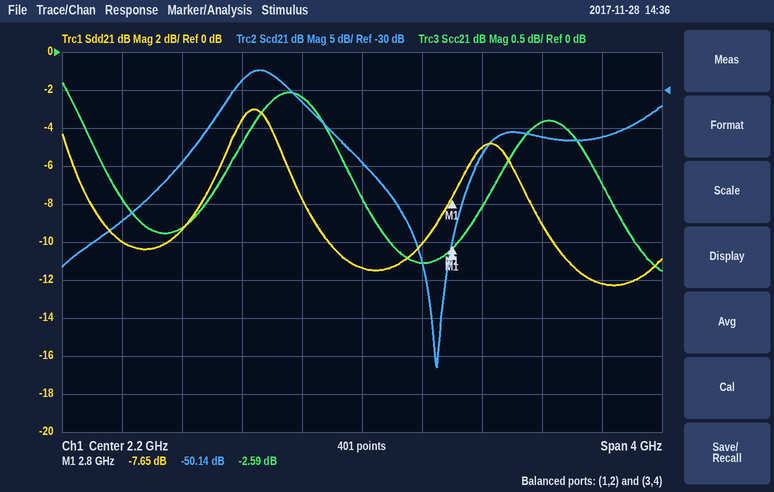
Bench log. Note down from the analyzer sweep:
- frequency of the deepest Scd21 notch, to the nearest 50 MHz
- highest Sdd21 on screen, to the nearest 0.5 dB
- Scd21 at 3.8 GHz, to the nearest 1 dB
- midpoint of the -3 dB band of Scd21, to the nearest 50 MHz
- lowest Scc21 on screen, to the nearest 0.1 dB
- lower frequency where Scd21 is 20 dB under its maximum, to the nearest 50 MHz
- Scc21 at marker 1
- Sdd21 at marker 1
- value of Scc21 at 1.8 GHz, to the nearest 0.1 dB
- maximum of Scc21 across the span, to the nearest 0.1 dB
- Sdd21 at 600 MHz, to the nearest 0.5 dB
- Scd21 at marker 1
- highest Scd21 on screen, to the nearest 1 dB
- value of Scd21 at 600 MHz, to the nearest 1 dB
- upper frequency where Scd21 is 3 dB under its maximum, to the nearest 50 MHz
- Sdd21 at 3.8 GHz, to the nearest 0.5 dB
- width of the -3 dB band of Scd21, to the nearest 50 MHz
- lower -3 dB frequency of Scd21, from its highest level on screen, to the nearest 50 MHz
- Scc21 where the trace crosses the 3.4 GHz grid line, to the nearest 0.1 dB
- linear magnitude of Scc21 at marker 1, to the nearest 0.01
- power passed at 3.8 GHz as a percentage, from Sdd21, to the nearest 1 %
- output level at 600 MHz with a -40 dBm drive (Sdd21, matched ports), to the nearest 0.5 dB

2.70 GHz
-3.0 dB
-36 dB
1.55 GHz
-2.9 dB
600 MHz
-2.59 dB
-7.65 dB
-0.6 dB
-0.4 dB
-10.0 dB
-50.14 dB
-27 dB
-47 dB
1.75 GHz
-12.0 dB
400 MHz
1.35 GHz
-0.9 dB
0.74
6 %
-50.0 dBm
